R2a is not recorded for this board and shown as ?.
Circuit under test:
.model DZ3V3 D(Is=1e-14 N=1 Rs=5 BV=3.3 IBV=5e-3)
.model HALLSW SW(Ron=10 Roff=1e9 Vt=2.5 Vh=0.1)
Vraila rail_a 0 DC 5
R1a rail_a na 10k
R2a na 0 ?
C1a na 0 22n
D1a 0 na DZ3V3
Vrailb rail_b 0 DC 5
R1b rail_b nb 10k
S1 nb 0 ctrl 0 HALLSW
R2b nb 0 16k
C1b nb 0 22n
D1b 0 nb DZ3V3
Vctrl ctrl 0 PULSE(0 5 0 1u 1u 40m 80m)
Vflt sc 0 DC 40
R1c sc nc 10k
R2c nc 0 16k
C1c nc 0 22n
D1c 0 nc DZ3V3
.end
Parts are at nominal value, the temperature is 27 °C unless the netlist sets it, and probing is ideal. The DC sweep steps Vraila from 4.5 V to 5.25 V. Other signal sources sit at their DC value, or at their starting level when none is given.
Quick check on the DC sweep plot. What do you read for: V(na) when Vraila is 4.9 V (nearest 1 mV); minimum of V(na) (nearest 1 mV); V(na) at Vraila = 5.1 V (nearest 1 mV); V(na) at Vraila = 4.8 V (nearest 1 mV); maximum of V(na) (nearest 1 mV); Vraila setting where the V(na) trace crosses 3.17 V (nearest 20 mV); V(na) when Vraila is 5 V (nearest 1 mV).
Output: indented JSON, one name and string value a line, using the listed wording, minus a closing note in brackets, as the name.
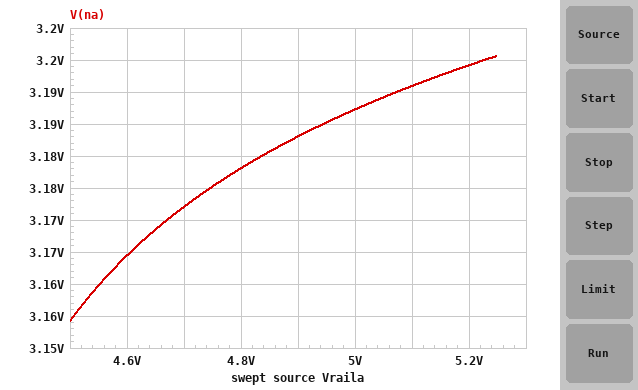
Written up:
{
  "V(na) when Vraila is 4.9 V": "3.183 V",
  "minimum of V(na)": "3.154 V",
  "V(na) at Vraila = 5.1 V": "3.191 V",
  "V(na) at Vraila = 4.8 V": "3.178 V",
  "maximum of V(na)": "3.196 V",
  "Vraila setting where the V(na) trace crosses 3.17 V": "4.60 V",
  "V(na) when Vraila is 5 V": "3.187 V"
}
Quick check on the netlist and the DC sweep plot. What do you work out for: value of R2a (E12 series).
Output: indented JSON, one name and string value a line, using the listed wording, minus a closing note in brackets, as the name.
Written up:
{
  "value of R2a": "27 kΩ"
}
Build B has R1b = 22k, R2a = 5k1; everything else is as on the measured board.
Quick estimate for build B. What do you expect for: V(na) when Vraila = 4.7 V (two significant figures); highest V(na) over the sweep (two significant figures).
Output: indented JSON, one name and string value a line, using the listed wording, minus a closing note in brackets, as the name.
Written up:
{
  "V(na) when Vraila = 4.7 V": "1.6 V",
  "highest V(na) over the sweep": "1.8 V"
}
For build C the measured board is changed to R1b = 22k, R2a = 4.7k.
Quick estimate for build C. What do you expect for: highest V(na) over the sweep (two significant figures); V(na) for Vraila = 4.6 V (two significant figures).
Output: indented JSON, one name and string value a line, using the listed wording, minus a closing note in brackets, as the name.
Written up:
{
  "highest V(na) over the sweep": "1.7 V",
  "V(na) for Vraila = 4.6 V": "1.5 V"
}
